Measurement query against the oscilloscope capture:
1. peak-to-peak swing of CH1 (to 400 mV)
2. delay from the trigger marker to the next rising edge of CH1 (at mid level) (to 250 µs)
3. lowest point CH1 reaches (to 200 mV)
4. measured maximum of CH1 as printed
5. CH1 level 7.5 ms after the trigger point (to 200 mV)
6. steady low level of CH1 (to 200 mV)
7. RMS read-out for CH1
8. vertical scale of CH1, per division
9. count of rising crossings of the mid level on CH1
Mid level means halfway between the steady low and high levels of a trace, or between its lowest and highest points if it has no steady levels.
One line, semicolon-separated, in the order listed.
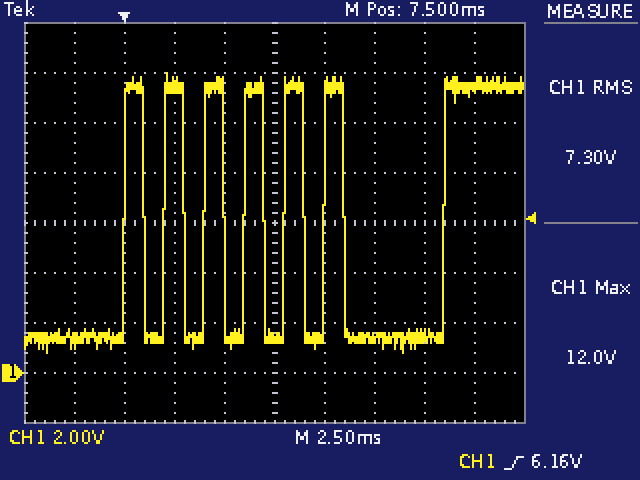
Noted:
11.2 V; 2.00 ms; 800 mV; 12.0 V; 1.4 V; 1.4 V; 7.30 V; 2 V; 7
